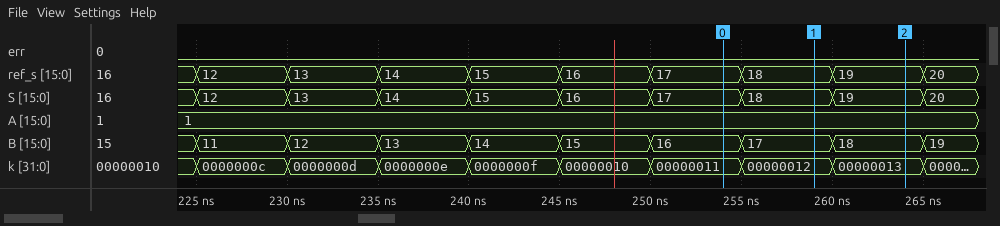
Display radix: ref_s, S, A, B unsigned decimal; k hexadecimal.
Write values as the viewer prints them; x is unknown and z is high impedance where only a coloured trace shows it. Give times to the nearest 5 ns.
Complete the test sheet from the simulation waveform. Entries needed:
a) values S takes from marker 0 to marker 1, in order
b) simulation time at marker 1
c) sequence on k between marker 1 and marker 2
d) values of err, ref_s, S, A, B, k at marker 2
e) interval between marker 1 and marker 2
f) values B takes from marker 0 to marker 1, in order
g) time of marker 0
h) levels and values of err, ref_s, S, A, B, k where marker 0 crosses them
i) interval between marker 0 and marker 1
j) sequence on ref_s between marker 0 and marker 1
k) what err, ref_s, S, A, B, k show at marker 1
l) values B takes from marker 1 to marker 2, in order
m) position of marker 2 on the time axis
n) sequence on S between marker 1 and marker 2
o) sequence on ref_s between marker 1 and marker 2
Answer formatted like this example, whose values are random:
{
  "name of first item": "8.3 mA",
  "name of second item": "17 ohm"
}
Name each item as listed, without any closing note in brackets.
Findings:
{
  "values S takes from marker 0 to marker 1, in order": "17, 18",
  "simulation time at marker 1": "260 ns",
  "sequence on k between marker 1 and marker 2": "00000012, 00000013",
  "values of err, ref_s, S, A, B, k at marker 2": "err=0, ref_s=19, S=19, A=1, B=18, k=00000013",
  "interval between marker 1 and marker 2": "5 ns",
  "values B takes from marker 0 to marker 1, in order": "16, 17",
  "time of marker 0": "255 ns",
  "levels and values of err, ref_s, S, A, B, k where marker 0 crosses them": "err=0, ref_s=17, S=17, A=1, B=16, k=00000011",
  "interval between marker 0 and marker 1": "5 ns",
  "sequence on ref_s between marker 0 and marker 1": "17, 18",
  "what err, ref_s, S, A, B, k show at marker 1": "err=0, ref_s=18, S=18, A=1, B=17, k=00000012",
  "values B takes from marker 1 to marker 2, in order": "17, 18",
  "position of marker 2 on the time axis": "265 ns",
  "sequence on S between marker 1 and marker 2": "18, 19",
  "sequence on ref_s between marker 1 and marker 2": "18, 19"
}
